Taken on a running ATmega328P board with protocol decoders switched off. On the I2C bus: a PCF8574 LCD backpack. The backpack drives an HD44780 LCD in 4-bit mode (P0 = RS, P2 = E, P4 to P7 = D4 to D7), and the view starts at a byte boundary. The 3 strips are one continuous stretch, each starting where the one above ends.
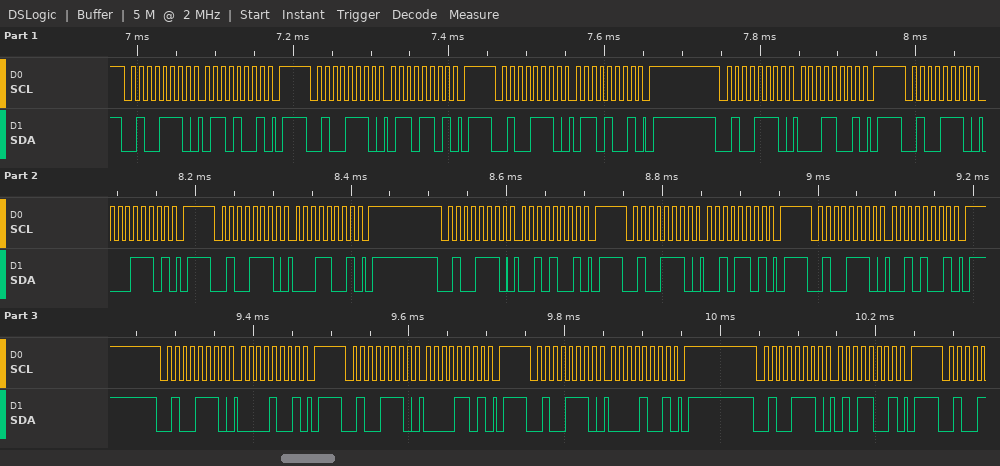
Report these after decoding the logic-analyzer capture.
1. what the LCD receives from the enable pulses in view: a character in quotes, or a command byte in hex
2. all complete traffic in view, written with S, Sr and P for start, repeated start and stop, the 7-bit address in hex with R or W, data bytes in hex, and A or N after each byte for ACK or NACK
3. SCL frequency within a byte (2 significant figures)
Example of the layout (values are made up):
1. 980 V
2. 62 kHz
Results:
1. 'a' ' '
2. S 27W A 69 A P S 27W A 6D A P S 27W A 69 A P S 27W A 19 A P S 27W A 1D A P S 27W A 19 A P S 27W A 29 A P S 27W A 2D A P S 27W A 29 A P S 27W A 09 A P S 27W A 0D A P S 27W A 09 A P S 27W A 59 A P
3. 100 kHz
